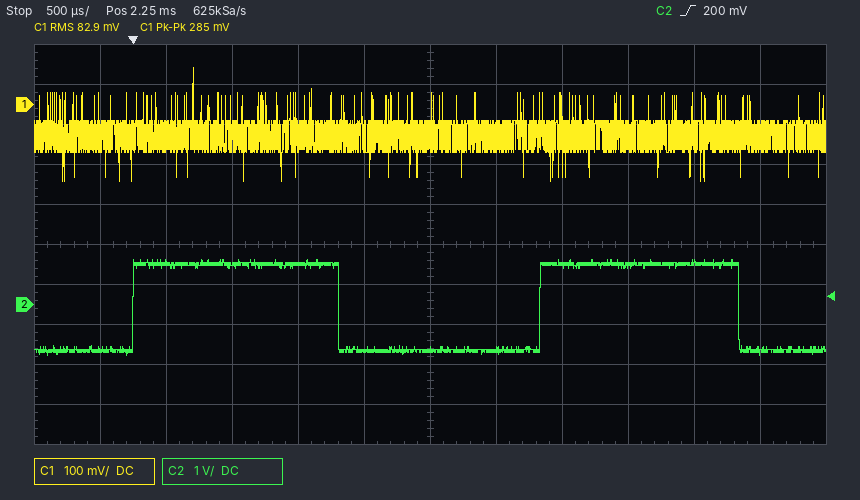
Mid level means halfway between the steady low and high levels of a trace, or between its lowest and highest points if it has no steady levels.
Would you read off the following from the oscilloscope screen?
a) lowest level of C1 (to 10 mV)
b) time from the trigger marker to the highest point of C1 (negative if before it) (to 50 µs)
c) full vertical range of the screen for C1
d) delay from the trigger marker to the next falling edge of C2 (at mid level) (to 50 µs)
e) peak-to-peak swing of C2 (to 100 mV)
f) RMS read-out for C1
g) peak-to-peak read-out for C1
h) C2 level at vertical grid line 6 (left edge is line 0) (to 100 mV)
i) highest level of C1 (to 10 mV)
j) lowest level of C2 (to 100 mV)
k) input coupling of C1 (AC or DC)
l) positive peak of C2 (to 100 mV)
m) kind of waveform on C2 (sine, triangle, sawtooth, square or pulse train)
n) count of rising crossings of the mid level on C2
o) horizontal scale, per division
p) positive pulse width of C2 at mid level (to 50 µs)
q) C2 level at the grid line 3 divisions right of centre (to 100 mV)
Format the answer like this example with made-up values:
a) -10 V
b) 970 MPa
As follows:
a) -190 mV
b) +450 µs
c) 1 V
d) 1.55 ms
e) 2.4 V
f) 82.9 mV
g) 285 mV
h) -1.1 V
i) 90 mV
j) -1.3 V
k) DC
l) 1.1 V
m) square
n) 2
o) 500 µs
p) 1.55 ms
q) 1.0 V
